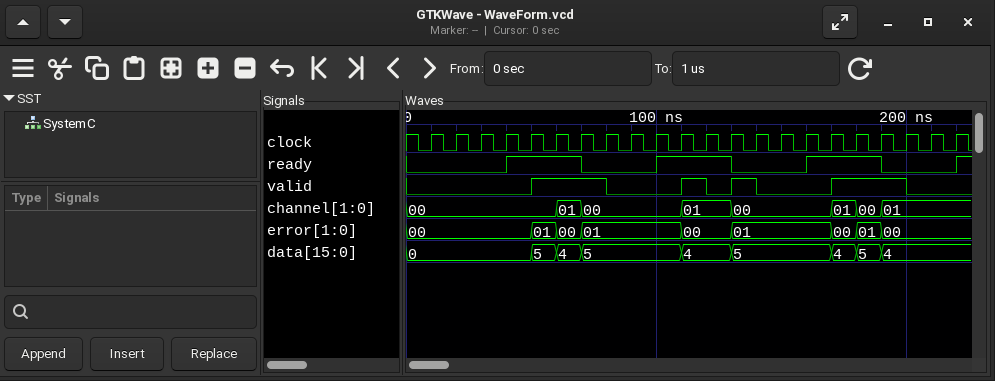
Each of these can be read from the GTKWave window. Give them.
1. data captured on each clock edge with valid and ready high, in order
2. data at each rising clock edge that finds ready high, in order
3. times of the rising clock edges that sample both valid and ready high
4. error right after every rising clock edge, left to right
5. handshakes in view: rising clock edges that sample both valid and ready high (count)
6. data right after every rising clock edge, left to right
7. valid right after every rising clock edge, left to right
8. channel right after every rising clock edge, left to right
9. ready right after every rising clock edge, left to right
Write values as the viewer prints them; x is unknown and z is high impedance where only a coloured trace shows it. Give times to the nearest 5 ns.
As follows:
5, 4, 4, 4, 5
0, 5, 4, 5, 4, 4, 5, 4, 5
60 ns, 70 ns, 120 ns, 180 ns, 190 ns
00, 00, 00, 00, 01, 00, 01, 01, 01, 01, 00, 00, 01, 01, 01, 01, 00, 01, 00, 00, 00, 00
5
0, 0, 0, 0, 5, 4, 5, 5, 5, 5, 4, 4, 5, 5, 5, 5, 4, 5, 4, 4, 4, 4
0 0 0 0 1 1 1 0 0 0 1 0 1 0 0 0 1 1 1 0 0 0
00, 00, 00, 00, 00, 01, 00, 00, 00, 00, 01, 01, 00, 00, 00, 00, 01, 00, 01, 01, 01, 01
0 0 0 1 1 1 0 0 0 1 1 1 0 0 0 1 1 1 0 0 0 1
